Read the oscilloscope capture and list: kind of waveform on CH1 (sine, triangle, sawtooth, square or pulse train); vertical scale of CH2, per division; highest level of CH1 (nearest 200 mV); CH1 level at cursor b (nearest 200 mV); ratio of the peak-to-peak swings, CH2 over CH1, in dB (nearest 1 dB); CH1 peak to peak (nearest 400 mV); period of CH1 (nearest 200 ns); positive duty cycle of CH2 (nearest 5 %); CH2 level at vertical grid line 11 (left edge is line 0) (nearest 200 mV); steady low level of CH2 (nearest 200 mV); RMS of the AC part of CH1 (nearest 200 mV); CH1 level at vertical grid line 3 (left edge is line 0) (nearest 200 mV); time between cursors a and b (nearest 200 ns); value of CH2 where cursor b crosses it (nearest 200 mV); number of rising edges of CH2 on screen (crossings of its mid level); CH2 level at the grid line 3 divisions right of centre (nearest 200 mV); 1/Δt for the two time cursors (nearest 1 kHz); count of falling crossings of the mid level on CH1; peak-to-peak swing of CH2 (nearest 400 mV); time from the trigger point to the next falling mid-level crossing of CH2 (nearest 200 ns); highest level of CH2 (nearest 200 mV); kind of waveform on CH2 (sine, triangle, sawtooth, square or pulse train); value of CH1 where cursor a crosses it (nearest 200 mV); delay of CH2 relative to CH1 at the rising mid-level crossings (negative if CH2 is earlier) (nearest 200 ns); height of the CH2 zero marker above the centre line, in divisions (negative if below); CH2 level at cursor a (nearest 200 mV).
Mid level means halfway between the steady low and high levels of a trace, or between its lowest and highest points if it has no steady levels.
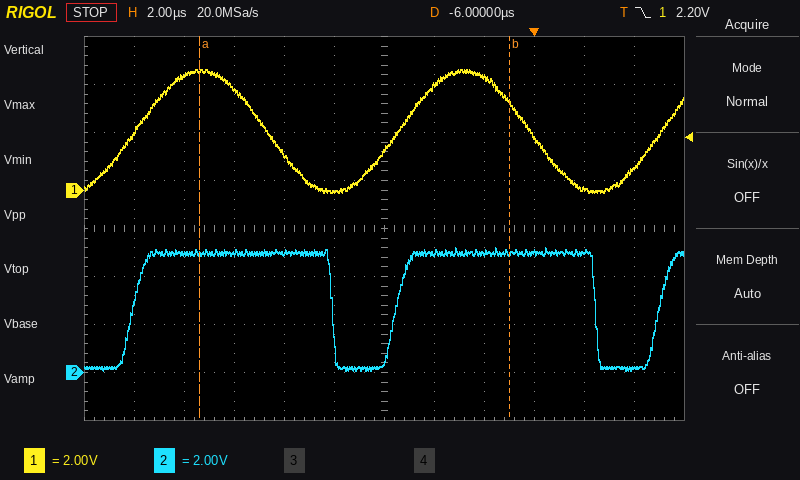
sine
2 V
5.0 V
3.6 V
0 dB
5.2 V
10.6 µs
75 %
200 mV
200 mV
1.8 V
4.2 V
12.4 µs
5.0 V
3
5.0 V
81 kHz
2
5.2 V
2.4 µs
5.2 V
pulse train
5.0 V
-200 ns
-3.0 div
5.0 V
